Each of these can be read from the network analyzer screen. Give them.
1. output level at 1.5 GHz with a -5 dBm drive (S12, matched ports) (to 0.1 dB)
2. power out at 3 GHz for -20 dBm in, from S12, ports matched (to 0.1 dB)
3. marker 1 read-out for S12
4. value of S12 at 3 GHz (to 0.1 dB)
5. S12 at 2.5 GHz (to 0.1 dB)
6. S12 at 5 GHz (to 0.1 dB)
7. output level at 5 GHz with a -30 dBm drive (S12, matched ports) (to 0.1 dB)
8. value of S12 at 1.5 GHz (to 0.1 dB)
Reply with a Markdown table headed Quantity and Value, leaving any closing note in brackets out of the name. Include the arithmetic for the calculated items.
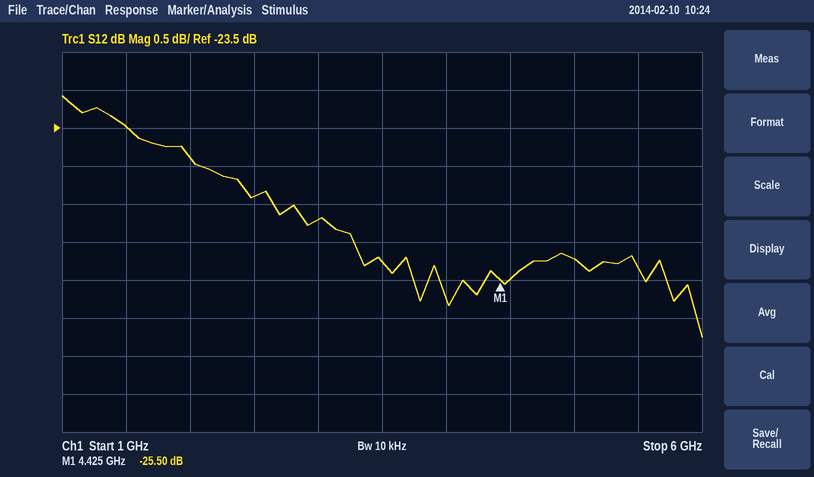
| Quantity | Value |
|---|---|
| output level at 1.5 GHz with a -5 dBm drive (S12, matched ports) | -5 dBm + (-23.5 dB) = -28.5 dBm |
| power out at 3 GHz for -20 dBm in, from S12, ports matched | -20 dBm + (-24.7 dB) = -44.7 dBm |
| marker 1 read-out for S12 | -25.50 dB |
| value of S12 at 3 GHz | -24.7 dB |
| S12 at 2.5 GHz | -24.4 dB |
| S12 at 5 GHz | -25.2 dB |
| output level at 5 GHz with a -30 dBm drive (S12, matched ports) | -30 dBm + (-25.2 dB) = -55.2 dBm |
| value of S12 at 1.5 GHz | -23.5 dB |
